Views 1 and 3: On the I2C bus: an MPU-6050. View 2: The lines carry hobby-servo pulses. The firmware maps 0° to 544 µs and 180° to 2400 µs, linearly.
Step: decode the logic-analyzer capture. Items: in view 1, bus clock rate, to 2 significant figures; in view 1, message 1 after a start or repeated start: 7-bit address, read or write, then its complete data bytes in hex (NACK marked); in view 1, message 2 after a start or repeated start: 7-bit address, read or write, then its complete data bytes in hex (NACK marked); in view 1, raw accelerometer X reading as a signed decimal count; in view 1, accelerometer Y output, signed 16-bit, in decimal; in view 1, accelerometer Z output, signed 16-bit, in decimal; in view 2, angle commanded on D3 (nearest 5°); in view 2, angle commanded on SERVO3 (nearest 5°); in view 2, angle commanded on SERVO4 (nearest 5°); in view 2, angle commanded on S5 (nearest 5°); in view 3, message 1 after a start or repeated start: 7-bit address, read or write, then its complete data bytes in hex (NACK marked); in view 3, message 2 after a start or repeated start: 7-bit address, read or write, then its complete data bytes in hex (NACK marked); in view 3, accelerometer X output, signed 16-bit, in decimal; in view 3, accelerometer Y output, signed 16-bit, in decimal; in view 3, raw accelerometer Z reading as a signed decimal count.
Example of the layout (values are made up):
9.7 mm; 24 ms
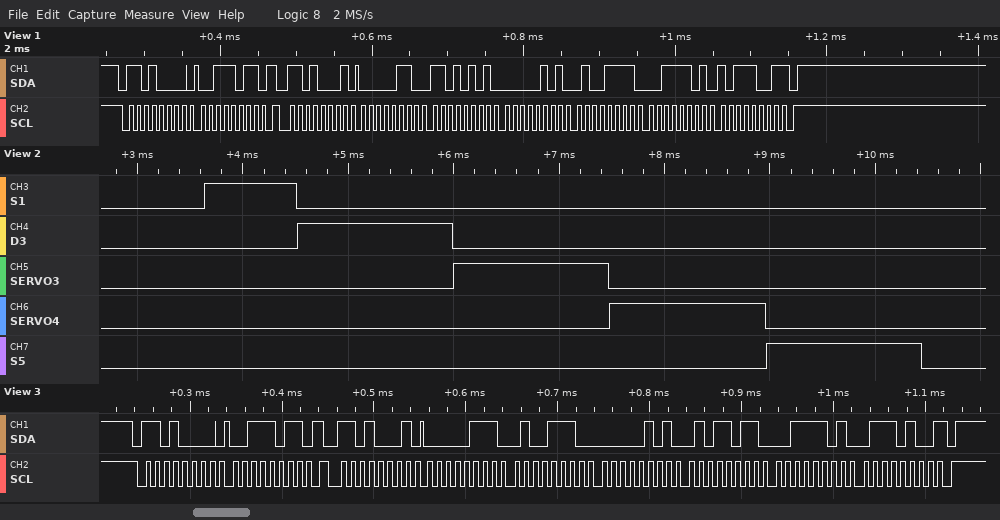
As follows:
100 kHz; 0x68 write: 3B; 0x68 read: 06 D5 05 4F 3D B9 NACK; 1749; 1359; 15801; 90°; 90°; 90°; 90°; 0x68 write: 3B; 0x68 read: 07 4E 05 5B 3D 74 NACK; 1870; 1371; 15732
